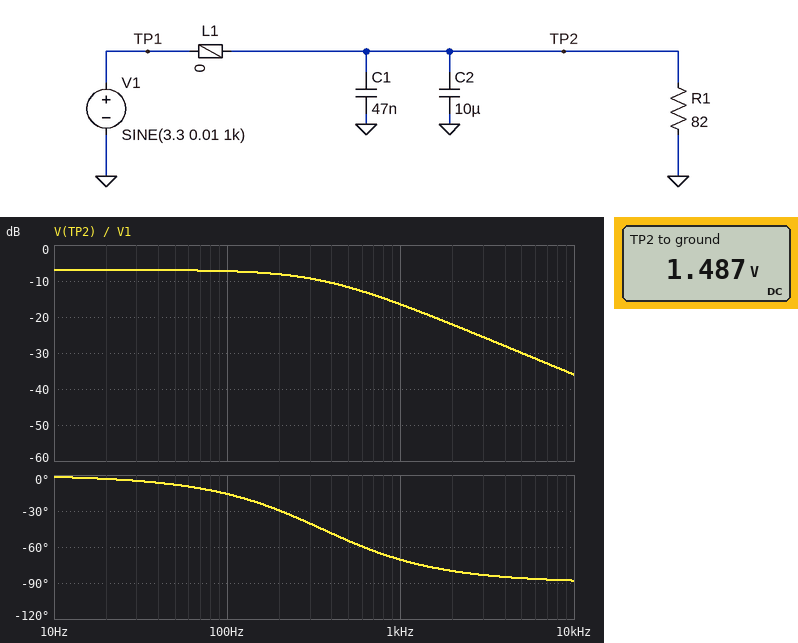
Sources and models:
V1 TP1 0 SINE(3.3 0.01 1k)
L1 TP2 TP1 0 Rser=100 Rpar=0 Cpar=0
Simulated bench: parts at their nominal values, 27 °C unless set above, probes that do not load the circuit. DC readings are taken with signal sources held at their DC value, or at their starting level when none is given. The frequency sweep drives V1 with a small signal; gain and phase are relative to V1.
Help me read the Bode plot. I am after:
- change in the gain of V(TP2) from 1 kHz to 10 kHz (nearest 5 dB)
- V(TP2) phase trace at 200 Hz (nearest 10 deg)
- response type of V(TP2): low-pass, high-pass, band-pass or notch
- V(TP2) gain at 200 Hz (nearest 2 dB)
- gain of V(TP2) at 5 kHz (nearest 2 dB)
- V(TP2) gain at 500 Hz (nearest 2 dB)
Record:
-20 dB
-30 deg
low-pass
-8 dB
-30 dB
-12 dB
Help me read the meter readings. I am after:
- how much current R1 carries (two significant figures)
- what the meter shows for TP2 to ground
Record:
18 mA
1.487 V
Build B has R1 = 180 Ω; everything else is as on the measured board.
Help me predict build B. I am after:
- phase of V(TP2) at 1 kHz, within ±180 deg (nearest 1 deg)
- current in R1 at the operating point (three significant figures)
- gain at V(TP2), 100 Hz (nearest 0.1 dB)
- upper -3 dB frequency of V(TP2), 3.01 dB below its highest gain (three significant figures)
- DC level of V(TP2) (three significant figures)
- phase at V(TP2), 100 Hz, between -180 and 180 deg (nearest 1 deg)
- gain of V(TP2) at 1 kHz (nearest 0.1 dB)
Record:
-76 deg
11.8 mA
-4.5 dB
246 Hz
2.12 V
-22 deg
-16.3 dB
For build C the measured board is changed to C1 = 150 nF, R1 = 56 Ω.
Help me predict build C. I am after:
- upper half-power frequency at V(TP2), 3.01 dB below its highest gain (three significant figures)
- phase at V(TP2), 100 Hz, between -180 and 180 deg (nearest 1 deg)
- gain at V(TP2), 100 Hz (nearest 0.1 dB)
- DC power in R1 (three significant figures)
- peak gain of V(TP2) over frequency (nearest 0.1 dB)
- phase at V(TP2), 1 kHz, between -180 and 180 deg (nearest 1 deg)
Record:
437 Hz
-13 deg
-9.1 dB
25.1 mW
-8.9 dB
-66 deg
